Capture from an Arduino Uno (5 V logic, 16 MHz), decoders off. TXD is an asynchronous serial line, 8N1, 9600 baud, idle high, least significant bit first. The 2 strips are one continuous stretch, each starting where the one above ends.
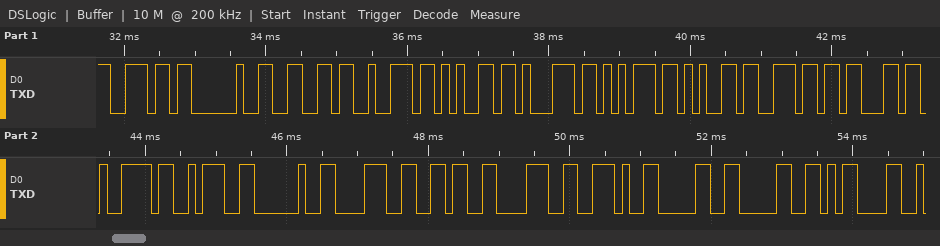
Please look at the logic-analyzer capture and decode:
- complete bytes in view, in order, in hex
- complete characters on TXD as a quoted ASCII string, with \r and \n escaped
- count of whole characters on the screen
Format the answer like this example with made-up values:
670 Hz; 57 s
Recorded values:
6E 20 66 72 65 71 75 65 6E 63 79 3A 20 38 36 38 2E 30 30 0D; "n frequency: 868.00\r"; 20
